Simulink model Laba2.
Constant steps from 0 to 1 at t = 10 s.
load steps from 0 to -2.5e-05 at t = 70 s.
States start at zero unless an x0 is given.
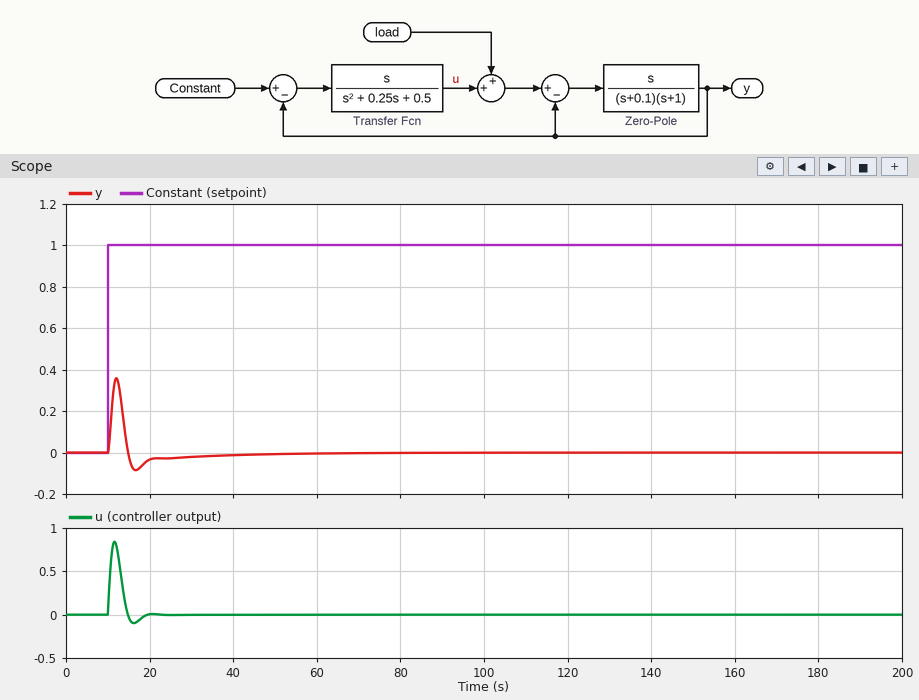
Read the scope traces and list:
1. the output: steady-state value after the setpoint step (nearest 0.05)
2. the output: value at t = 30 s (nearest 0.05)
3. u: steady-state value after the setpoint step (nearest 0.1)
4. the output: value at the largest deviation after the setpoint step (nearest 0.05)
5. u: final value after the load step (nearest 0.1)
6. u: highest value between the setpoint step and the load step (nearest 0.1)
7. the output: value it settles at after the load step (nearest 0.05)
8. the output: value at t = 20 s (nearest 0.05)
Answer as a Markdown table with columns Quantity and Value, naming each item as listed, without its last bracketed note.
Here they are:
| Quantity | Value |
|---|---|
| the output: steady-state value after the setpoint step | 0.00 |
| the output: value at t = 30 s | 0.00 |
| u: steady-state value after the setpoint step | 0.0 |
| the output: value at the largest deviation after the setpoint step | 0.35 |
| u: final value after the load step | 0.0 |
| u: highest value between the setpoint step and the load step | 0.8 |
| the output: value it settles at after the load step | 0.00 |
| the output: value at t = 20 s | -0.05 |
